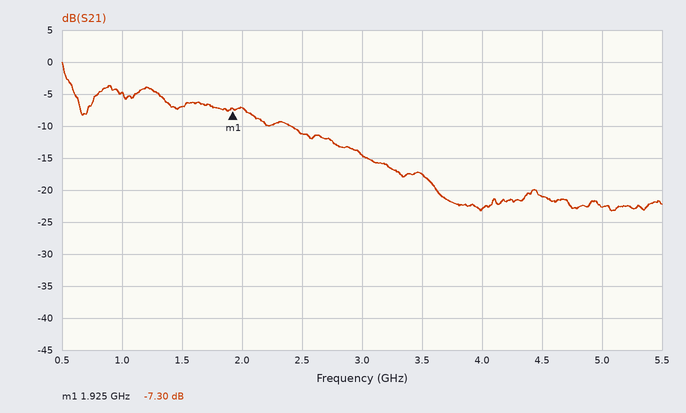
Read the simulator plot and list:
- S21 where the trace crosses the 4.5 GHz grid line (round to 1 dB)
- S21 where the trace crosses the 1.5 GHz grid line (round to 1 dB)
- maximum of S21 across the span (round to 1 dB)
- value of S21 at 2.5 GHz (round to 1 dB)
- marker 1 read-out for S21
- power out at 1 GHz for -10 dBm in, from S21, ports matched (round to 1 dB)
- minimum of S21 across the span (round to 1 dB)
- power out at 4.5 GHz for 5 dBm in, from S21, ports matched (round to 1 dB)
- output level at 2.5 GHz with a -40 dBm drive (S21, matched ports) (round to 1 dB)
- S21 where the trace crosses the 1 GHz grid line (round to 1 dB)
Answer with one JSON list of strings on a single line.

["-21 dB", "-7 dB", "0 dB", "-11 dB", "-7.30 dB", "-15 dBm", "-23 dB", "-16 dBm", "-51 dBm", "-5 dB"]
